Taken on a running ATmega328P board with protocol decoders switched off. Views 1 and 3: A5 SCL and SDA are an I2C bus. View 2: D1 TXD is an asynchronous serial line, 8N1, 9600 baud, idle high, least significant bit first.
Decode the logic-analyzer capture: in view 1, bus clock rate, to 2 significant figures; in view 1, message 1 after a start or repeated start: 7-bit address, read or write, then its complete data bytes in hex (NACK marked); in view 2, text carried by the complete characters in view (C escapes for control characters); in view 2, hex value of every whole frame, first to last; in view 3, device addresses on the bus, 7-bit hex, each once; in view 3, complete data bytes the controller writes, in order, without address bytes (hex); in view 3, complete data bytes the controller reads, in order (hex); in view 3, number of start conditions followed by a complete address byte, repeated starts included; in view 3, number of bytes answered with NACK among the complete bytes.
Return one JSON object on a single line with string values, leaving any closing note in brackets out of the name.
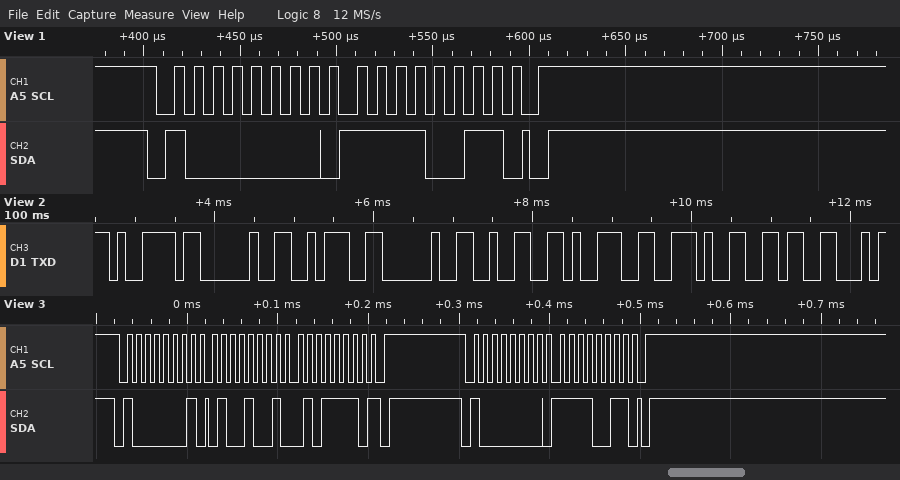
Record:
{"in view 1, bus clock rate, to 2 significant figures": "100 kHz", "in view 1, message 1 after a start or repeated start: 7-bit address, read or write, then its complete data bytes in hex": "0x40 write: F3", "in view 2, text carried by the complete characters in view": "\"y : 29.6\"", "in view 2, hex value of every whole frame, first to last": "79 20 3A 20 32 39 2E 36", "in view 3, device addresses on the bus, 7-bit hex, each once": "0x40", "in view 3, complete data bytes the controller writes, in order, without address bytes": "F3", "in view 3, complete data bytes the controller reads, in order": "49 5E", "in view 3, number of start conditions followed by a complete address byte, repeated starts included": "2", "in view 3, number of bytes answered with NACK among the complete bytes": "1"}
